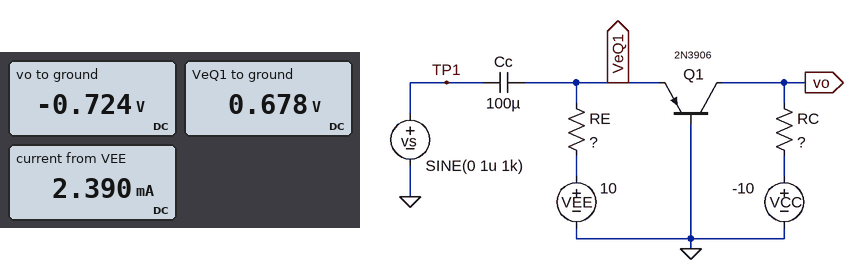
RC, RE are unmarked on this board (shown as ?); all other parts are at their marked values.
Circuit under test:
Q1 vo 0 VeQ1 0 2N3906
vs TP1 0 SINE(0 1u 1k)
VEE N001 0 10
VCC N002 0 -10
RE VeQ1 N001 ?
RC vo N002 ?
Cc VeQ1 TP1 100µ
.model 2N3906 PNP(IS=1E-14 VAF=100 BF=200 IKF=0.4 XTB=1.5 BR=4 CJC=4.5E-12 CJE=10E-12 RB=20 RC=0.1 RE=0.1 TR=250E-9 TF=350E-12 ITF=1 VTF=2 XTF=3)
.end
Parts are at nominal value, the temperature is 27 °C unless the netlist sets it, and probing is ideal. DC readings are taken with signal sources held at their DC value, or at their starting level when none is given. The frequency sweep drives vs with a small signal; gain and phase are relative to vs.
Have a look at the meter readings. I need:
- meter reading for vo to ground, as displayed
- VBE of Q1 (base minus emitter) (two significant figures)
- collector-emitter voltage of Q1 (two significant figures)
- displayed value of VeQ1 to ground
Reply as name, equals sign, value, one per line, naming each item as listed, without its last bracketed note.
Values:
meter reading for vo to ground, as displayed = -0.724 V
VBE of Q1 (base minus emitter) = -680 mV
collector-emitter voltage of Q1 = -1.4 V
displayed value of VeQ1 to ground = 0.678 V
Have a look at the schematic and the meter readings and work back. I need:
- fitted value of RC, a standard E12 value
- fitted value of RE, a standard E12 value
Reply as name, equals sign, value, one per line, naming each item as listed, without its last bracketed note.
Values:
fitted value of RC, a standard E12 value = 3.9 kΩ
fitted value of RE, a standard E12 value = 3.9 kΩ
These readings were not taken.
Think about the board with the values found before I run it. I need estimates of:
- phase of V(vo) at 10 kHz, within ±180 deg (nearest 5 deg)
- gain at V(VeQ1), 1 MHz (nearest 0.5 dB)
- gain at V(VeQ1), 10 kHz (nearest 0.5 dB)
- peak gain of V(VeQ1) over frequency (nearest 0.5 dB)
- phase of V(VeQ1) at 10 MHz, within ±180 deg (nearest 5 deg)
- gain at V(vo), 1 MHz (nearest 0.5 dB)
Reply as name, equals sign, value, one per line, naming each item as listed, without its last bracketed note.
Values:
phase of V(vo) at 10 kHz, within ±180 deg = 0 deg
gain at V(VeQ1), 1 MHz = 0 dB
gain at V(VeQ1), 10 kHz = 0 dB
peak gain of V(VeQ1) over frequency = 0 dB
phase of V(VeQ1) at 10 MHz, within ±180 deg = 0 deg
gain at V(vo), 1 MHz = 50.0 dB
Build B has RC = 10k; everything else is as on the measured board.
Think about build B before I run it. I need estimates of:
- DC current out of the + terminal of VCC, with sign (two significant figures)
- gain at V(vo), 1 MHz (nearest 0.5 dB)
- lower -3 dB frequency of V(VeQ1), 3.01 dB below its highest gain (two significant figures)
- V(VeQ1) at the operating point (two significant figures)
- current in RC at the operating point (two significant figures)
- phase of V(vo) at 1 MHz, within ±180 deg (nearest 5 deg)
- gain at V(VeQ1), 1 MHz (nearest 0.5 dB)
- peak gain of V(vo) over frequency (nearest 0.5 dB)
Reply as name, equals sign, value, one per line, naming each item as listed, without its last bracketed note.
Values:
DC current out of the + terminal of VCC, with sign = -1.1 mA
gain at V(vo), 1 MHz = -1.5 dB
lower -3 dB frequency of V(VeQ1), 3.01 dB below its highest gain = 43 Hz
V(VeQ1) at the operating point = 730 mV
current in RC at the operating point = 1.1 mA
phase of V(vo) at 1 MHz, within ±180 deg = -5 deg
gain at V(VeQ1), 1 MHz = 0 dB
peak gain of V(vo) over frequency = 0.5 dB
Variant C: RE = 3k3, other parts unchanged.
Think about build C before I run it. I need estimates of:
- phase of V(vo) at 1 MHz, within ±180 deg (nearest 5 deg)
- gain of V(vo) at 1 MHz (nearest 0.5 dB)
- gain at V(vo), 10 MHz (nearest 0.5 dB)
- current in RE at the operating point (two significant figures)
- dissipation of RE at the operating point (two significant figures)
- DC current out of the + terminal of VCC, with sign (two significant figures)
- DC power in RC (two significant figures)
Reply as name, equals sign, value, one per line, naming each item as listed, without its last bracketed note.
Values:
phase of V(vo) at 1 MHz, within ±180 deg = -50 deg
gain of V(vo) at 1 MHz = 5.5 dB
gain at V(vo), 10 MHz = -3.0 dB
current in RE at the operating point = 2.8 mA
dissipation of RE at the operating point = 26 mW
DC current out of the + terminal of VCC, with sign = -2.7 mA
DC power in RC = 29 mW
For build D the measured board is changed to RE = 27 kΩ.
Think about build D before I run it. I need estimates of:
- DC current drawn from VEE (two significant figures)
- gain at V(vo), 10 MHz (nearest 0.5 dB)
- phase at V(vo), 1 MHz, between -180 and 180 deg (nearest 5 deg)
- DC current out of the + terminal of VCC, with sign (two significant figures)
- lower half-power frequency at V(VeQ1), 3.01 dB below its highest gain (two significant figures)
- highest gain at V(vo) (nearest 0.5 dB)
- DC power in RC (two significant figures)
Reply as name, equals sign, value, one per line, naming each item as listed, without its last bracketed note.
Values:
DC current drawn from VEE = 350 µA
gain at V(vo), 10 MHz = 33.0 dB
phase at V(vo), 1 MHz, between -180 and 180 deg = -5 deg
DC current out of the + terminal of VCC, with sign = -350 µA
lower half-power frequency at V(VeQ1), 3.01 dB below its highest gain = 21 Hz
highest gain at V(vo) = 34.0 dB
DC power in RC = 470 µW
